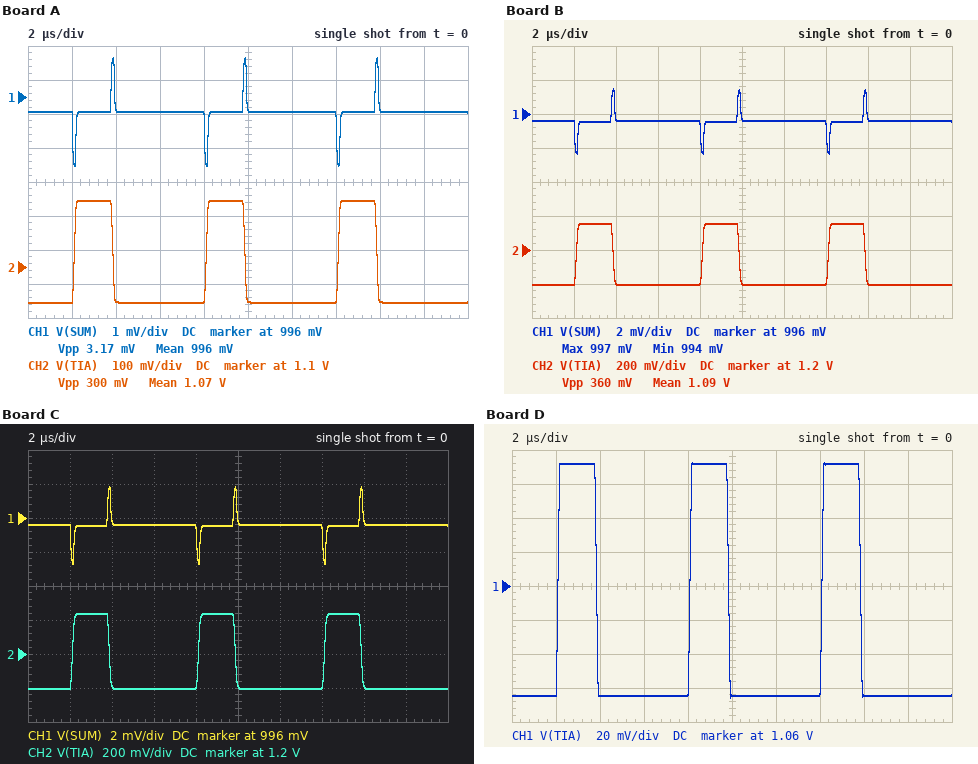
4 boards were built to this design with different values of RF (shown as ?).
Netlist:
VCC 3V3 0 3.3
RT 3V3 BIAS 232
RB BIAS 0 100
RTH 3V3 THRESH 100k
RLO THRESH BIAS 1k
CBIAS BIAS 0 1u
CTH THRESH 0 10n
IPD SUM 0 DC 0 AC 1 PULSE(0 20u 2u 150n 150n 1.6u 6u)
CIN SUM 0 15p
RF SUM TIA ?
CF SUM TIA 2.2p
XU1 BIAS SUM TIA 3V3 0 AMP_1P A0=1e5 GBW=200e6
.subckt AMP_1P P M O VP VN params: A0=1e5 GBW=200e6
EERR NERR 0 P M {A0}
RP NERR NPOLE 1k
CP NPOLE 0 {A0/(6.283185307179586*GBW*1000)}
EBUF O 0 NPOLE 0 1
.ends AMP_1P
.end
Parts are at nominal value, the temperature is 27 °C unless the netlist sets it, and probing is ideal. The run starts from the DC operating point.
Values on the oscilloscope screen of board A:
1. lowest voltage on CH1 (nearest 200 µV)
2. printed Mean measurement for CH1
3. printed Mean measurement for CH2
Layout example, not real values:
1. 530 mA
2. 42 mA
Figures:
1. 994.0 mV
2. 996 mV
3. 1.07 V
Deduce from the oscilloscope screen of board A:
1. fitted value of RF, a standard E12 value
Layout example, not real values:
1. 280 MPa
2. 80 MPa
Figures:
1. 15 kΩ
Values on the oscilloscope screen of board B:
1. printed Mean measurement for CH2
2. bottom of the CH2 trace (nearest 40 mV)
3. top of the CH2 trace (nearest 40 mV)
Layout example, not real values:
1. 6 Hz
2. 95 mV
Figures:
1. 1.09 V
2. 1.00 V
3. 1.36 V
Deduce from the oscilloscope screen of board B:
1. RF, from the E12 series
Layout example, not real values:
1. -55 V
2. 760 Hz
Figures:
1. 18 kΩ
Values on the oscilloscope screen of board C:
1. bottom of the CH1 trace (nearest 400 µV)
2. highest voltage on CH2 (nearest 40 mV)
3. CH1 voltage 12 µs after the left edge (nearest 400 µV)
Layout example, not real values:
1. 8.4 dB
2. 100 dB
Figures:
1. 993.2 mV
2. 1.44 V
3. 995.6 mV
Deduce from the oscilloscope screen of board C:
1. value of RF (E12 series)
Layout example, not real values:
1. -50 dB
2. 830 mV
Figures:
1. 22 kΩ
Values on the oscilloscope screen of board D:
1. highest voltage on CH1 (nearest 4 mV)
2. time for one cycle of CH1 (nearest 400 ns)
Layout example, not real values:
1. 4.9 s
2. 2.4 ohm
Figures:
1. 1.132 V
2. 6.0 µs
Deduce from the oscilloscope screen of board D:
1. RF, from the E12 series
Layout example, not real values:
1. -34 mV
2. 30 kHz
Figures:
1. 6.8 kΩ
